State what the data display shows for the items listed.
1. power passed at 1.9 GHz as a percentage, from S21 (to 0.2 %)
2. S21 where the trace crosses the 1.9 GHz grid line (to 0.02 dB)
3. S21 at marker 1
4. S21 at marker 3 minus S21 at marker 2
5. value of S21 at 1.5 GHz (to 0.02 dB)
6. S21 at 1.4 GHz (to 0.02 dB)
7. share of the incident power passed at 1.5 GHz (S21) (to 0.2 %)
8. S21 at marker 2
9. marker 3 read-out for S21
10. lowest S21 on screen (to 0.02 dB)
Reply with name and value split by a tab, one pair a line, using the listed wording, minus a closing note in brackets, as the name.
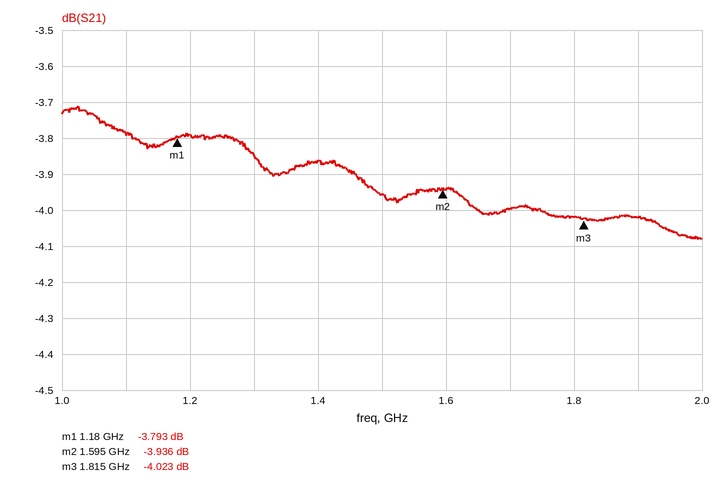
power passed at 1.9 GHz as a percentage, from S21	39.6 %
S21 where the trace crosses the 1.9 GHz grid line	-4.02 dB
S21 at marker 1	-3.793 dB
S21 at marker 3 minus S21 at marker 2	-0.087 dB
value of S21 at 1.5 GHz	-3.96 dB
S21 at 1.4 GHz	-3.86 dB
share of the incident power passed at 1.5 GHz (S21)	40.2 %
S21 at marker 2	-3.936 dB
marker 3 read-out for S21	-4.023 dB
lowest S21 on screen	-4.08 dB
